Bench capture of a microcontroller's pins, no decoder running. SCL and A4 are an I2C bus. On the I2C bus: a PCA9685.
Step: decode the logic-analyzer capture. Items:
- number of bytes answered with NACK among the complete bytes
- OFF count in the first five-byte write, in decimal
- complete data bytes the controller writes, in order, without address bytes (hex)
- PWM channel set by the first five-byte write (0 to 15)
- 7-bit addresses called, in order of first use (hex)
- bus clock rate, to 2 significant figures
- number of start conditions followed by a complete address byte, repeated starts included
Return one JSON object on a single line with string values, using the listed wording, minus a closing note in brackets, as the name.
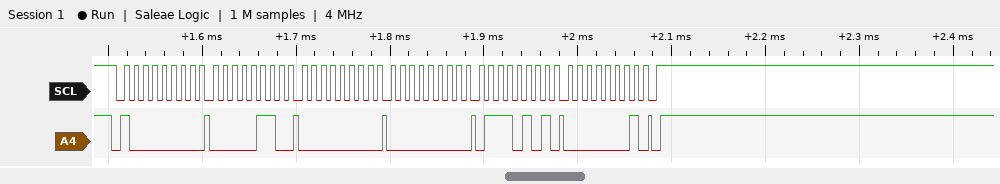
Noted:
{"number of bytes answered with NACK among the complete bytes": "0", "OFF count in the first five-byte write, in decimal": "373", "complete data bytes the controller writes, in order, without address bytes": "06 00 00 75 01", "PWM channel set by the first five-byte write": "0", "7-bit addresses called, in order of first use": "0x40", "bus clock rate, to 2 significant figures": "100 kHz", "number of start conditions followed by a complete address byte, repeated starts included": "1"}
